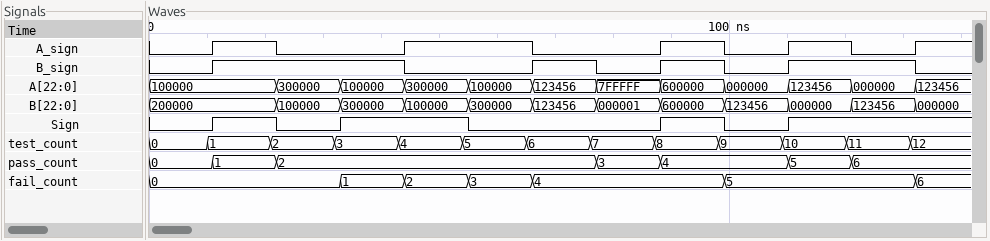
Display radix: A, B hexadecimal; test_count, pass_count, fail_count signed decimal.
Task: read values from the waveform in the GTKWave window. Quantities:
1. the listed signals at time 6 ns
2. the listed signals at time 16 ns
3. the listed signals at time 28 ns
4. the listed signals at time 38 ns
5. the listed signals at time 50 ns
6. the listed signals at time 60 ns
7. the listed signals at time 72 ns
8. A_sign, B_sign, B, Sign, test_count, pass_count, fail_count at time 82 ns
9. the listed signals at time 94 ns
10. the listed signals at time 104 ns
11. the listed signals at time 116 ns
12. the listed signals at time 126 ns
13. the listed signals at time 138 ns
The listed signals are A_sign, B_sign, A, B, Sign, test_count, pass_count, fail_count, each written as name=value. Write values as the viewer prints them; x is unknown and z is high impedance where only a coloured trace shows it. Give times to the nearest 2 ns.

A_sign=0, B_sign=0, A=100000, B=200000, Sign=0, test_count=0, pass_count=0, fail_count=0
A_sign=1, B_sign=1, A=100000, B=200000, Sign=1, test_count=1, pass_count=1, fail_count=0
A_sign=0, B_sign=1, A=300000, B=100000, Sign=0, test_count=2, pass_count=2, fail_count=0
A_sign=0, B_sign=1, A=100000, B=300000, Sign=1, test_count=3, pass_count=2, fail_count=1
A_sign=1, B_sign=0, A=300000, B=100000, Sign=1, test_count=4, pass_count=2, fail_count=2
A_sign=1, B_sign=0, A=100000, B=300000, Sign=0, test_count=5, pass_count=2, fail_count=3
A_sign=0, B_sign=1, A=123456, B=123456, Sign=0, test_count=6, pass_count=2, fail_count=4
A_sign=0, B_sign=0, B=000001, Sign=0, test_count=7, pass_count=3, fail_count=4
A_sign=1, B_sign=1, A=600000, B=600000, Sign=1, test_count=8, pass_count=4, fail_count=4
A_sign=0, B_sign=0, A=000000, B=123456, Sign=0, test_count=9, pass_count=4, fail_count=5
A_sign=1, B_sign=1, A=123456, B=000000, Sign=1, test_count=10, pass_count=5, fail_count=5
A_sign=0, B_sign=1, A=000000, B=123456, Sign=1, test_count=11, pass_count=6, fail_count=5
A_sign=1, B_sign=0, A=123456, B=000000, Sign=1, test_count=12, pass_count=6, fail_count=6
